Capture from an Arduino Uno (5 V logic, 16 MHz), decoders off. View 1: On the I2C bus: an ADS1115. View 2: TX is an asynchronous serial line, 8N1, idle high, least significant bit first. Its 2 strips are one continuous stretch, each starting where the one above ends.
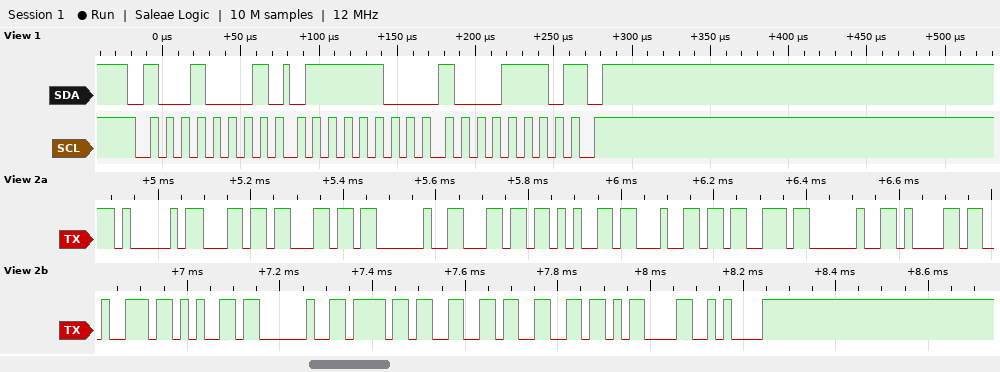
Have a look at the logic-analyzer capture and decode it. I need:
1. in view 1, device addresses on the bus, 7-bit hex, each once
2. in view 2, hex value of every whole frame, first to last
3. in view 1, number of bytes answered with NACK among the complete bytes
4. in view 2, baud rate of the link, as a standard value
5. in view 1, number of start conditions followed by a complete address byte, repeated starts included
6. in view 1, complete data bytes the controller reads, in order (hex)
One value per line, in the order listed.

0x48
0x41 0x6C 0x6C 0x20 0x6C 0x65 0x64 0x73 0x20 0x61 0x72 0x65 0x20 0x6F 0x66 0x66 0x0D 0x0A
1
57600 baud
1
7C 8E
